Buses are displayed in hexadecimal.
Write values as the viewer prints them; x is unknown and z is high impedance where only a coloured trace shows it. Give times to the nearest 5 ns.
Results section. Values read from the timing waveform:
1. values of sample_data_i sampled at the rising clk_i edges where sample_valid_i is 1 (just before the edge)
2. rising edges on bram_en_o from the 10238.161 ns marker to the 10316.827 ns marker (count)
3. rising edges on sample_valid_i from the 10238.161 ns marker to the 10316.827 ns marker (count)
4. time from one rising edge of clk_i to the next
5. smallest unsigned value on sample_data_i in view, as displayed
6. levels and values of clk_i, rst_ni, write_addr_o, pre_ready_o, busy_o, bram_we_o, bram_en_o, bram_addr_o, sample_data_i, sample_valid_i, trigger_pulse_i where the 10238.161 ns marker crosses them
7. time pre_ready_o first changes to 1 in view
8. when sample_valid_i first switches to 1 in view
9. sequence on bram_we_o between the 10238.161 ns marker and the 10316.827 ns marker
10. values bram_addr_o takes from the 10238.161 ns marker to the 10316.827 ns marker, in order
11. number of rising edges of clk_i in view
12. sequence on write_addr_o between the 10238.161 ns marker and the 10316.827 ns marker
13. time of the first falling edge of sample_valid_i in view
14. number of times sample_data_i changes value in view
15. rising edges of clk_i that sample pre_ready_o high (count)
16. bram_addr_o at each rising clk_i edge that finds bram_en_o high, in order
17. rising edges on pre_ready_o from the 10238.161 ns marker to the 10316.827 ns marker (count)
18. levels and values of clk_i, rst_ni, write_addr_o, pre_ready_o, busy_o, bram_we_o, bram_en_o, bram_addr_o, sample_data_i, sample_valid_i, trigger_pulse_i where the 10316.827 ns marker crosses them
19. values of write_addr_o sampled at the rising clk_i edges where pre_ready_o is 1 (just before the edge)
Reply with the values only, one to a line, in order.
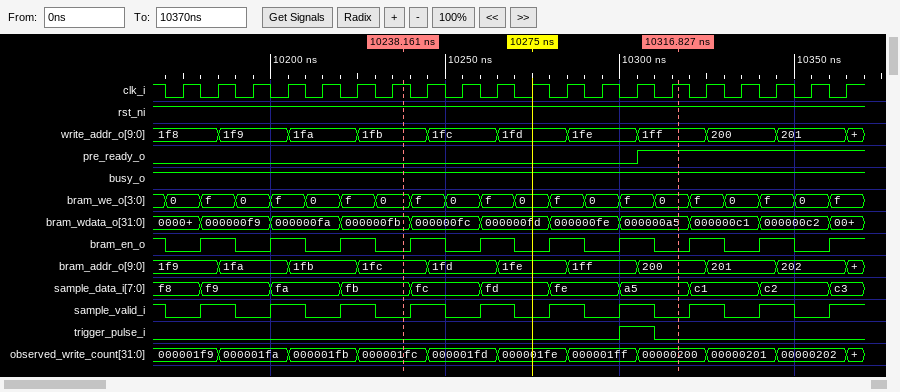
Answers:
f9, fa, fb, fc, fd, fe, a5, c1, c2, c3
4
4
10 ns
a5
clk_i=1, rst_ni=1, write_addr_o=1fb, pre_ready_o=0, busy_o=1, bram_we_o=0, bram_en_o=0, bram_addr_o=1fc, sample_data_i=fb, sample_valid_i=0, trigger_pulse_i=0
10305 ns
10180 ns
0, f, 0, f, 0, f, 0, f, 0
1fc, 1fd, 1fe, 1ff, 200
20
1fb, 1fc, 1fd, 1fe, 1ff
10170 ns
10
6
1f9, 1fa, 1fb, 1fc, 1fd, 1fe, 1ff, 200, 201, 202
1
clk_i=1, rst_ni=1, write_addr_o=1ff, pre_ready_o=1, busy_o=1, bram_we_o=0, bram_en_o=0, bram_addr_o=200, sample_data_i=a5, sample_valid_i=0, trigger_pulse_i=0
1ff, 1ff, 200, 200, 201, 201
